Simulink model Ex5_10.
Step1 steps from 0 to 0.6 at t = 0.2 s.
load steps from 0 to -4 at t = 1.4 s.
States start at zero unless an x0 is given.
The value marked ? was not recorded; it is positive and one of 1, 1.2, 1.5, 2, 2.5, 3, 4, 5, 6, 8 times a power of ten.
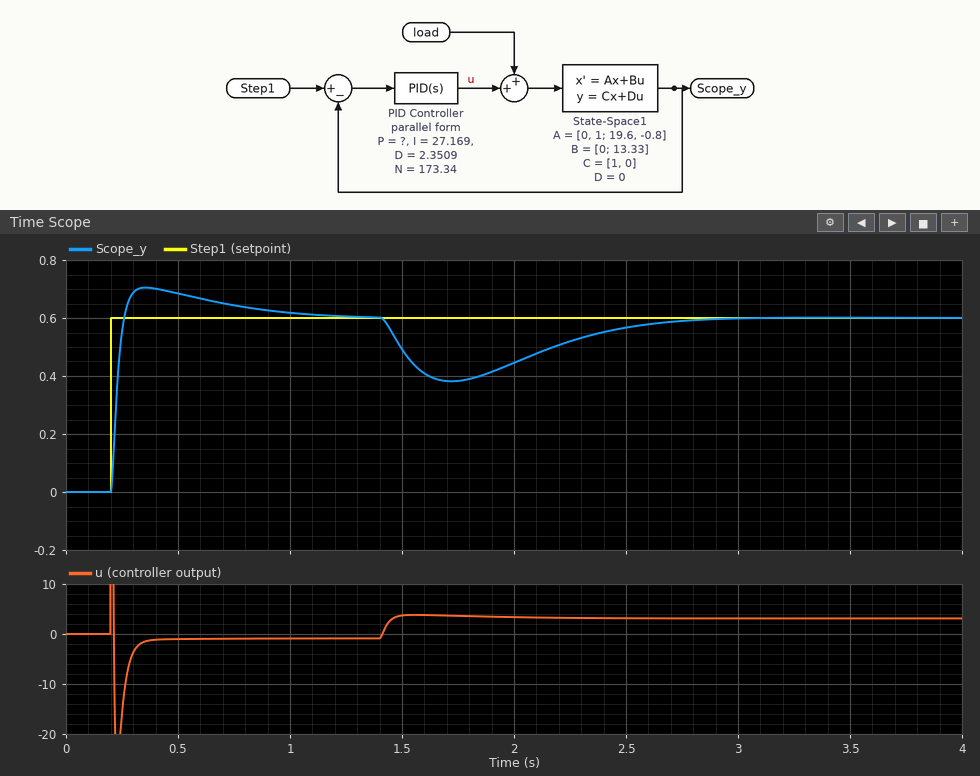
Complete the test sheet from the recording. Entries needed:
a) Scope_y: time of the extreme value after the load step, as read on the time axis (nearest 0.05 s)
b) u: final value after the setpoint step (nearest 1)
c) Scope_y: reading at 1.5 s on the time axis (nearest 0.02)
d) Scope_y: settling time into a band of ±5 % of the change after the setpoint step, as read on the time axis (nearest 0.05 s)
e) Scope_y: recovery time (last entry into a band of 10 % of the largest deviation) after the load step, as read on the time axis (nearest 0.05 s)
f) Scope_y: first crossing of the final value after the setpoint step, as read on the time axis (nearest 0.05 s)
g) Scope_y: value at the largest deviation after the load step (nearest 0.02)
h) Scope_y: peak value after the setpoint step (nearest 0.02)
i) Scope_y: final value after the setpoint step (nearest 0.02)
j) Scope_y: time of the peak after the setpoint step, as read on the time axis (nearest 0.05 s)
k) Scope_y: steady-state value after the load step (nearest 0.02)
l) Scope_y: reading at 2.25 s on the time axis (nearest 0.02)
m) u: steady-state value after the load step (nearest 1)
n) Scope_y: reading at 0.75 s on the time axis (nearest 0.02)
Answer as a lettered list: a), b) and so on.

a) 1.70 s
b) -1
c) 0.50
d) 0.85 s
e) 2.60 s
f) 0.25 s
g) 0.38
h) 0.70
i) 0.60
j) 0.35 s
k) 0.60
l) 0.52
m) 3
n) 0.64
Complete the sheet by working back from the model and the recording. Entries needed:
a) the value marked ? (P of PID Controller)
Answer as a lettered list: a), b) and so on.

a) 15
